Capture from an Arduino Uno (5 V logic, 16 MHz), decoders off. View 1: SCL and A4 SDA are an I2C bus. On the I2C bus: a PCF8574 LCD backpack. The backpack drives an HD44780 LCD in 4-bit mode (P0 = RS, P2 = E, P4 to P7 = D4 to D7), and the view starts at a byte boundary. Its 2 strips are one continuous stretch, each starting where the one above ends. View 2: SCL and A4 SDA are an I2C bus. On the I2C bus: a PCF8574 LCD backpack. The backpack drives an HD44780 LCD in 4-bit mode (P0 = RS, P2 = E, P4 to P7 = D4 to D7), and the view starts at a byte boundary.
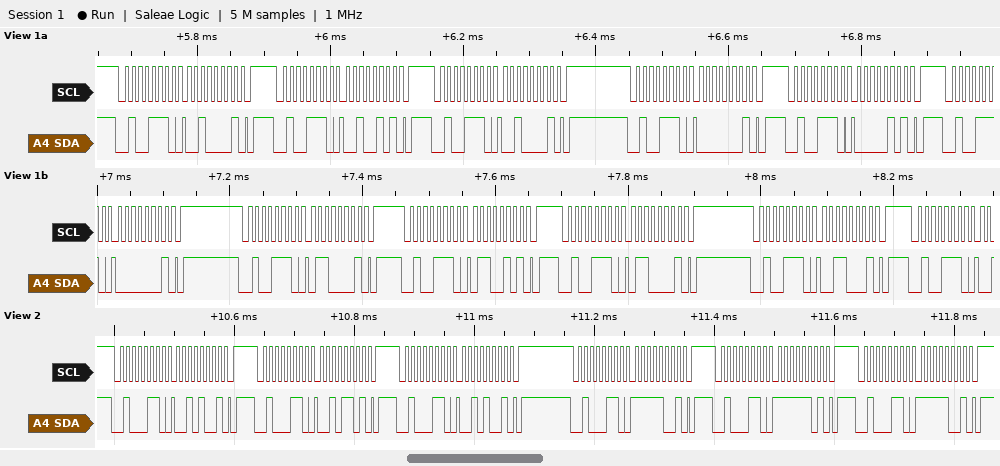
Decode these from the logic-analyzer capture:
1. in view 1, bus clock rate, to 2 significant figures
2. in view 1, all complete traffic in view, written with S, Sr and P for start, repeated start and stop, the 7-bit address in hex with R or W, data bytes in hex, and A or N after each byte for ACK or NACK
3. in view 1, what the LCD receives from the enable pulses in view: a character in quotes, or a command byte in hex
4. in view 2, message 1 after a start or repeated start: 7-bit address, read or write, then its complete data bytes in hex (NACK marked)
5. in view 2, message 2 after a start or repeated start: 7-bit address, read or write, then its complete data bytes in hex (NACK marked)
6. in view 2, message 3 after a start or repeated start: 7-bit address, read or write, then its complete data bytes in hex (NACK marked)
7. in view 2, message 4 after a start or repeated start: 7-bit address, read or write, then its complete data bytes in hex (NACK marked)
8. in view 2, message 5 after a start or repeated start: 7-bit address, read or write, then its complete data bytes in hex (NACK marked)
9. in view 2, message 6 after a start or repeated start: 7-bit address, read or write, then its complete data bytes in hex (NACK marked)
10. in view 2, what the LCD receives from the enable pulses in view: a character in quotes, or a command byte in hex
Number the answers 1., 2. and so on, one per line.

1. 100 kHz
2. S 27W A 21 A P S 27W A 25 A P S 27W A 21 A P S 27W A 01 A P S 27W A 05 A P S 27W A 01 A P S 27W A 61 A P S 27W A 65 A P S 27W A 61 A P S 27W A 31 A P S 27W A
3. ' '
4. 0x23 write: 29
5. 0x23 write: 2D
6. 0x23 write: 29
7. 0x23 write: F9
8. 0x23 write: FD
9. 0x23 write: F9
10. '/'
